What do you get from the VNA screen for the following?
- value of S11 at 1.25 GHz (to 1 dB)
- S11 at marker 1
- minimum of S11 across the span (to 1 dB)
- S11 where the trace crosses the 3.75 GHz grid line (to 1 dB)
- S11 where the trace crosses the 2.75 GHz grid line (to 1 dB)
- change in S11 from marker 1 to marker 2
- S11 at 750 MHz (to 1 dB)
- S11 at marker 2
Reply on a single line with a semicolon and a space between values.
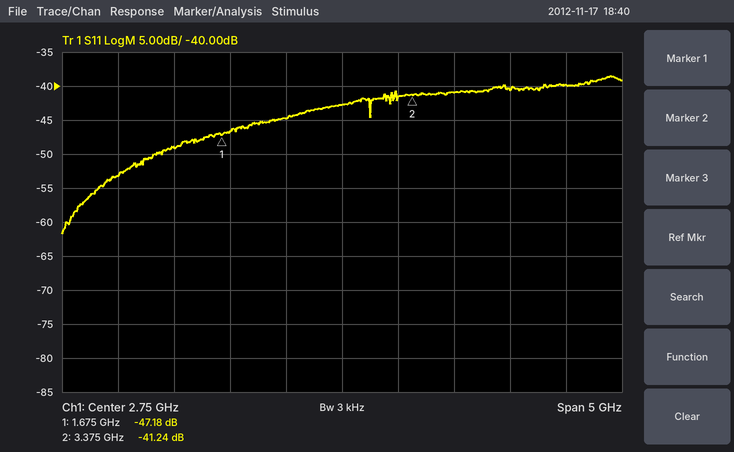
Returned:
-49 dB; -47.18 dB; -62 dB; -41 dB; -43 dB; 5.94 dB; -53 dB; -41.24 dB
